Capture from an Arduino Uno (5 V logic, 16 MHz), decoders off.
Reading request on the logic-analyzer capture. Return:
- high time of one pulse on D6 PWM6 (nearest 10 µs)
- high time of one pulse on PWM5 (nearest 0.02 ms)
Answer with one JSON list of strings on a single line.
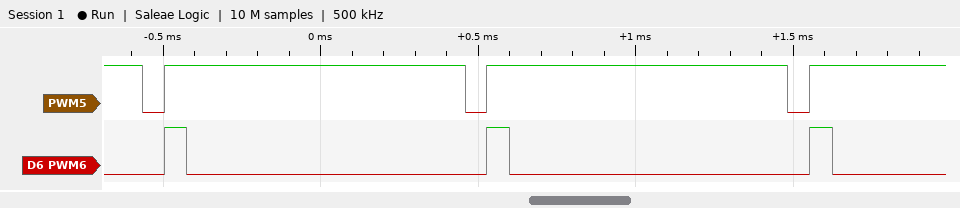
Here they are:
["70 µs", "0.96 ms"]
